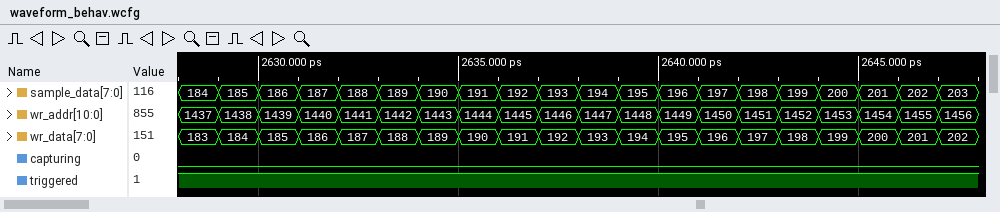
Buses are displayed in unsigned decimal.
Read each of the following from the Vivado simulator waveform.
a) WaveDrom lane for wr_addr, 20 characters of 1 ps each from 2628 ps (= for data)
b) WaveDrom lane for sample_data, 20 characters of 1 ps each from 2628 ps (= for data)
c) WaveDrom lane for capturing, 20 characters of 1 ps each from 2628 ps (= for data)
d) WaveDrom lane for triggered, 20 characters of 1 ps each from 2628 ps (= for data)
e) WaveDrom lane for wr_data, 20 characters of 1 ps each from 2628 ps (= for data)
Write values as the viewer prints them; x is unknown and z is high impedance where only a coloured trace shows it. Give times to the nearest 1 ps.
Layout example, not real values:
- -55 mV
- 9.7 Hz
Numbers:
- {name: 'wr_addr', wave: '====================', data: '1437 1438 1439 1440 1441 1442 1443 1444 1445 1446 1447 1448 1449 1450 1451 1452 1453 1454 1455 1456'}
- {name: 'sample_data', wave: '====================', data: '184 185 186 187 188 189 190 191 192 193 194 195 196 197 198 199 200 201 202 203'}
- {name: 'capturing', wave: '0...................'}
- {name: 'triggered', wave: '1...................'}
- {name: 'wr_data', wave: '====================', data: '183 184 185 186 187 188 189 190 191 192 193 194 195 196 197 198 199 200 201 202'}
